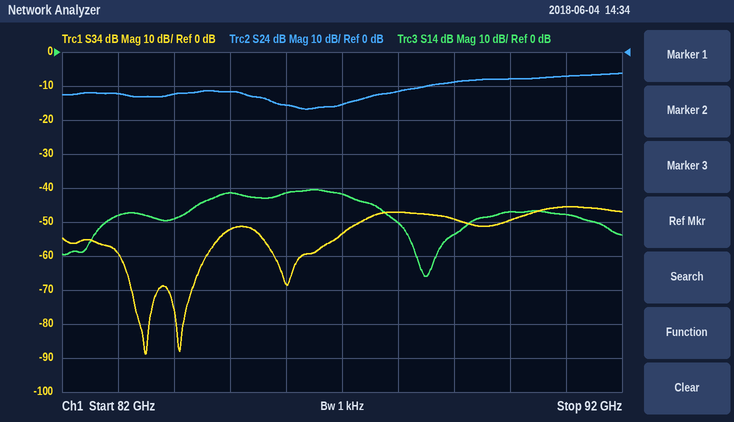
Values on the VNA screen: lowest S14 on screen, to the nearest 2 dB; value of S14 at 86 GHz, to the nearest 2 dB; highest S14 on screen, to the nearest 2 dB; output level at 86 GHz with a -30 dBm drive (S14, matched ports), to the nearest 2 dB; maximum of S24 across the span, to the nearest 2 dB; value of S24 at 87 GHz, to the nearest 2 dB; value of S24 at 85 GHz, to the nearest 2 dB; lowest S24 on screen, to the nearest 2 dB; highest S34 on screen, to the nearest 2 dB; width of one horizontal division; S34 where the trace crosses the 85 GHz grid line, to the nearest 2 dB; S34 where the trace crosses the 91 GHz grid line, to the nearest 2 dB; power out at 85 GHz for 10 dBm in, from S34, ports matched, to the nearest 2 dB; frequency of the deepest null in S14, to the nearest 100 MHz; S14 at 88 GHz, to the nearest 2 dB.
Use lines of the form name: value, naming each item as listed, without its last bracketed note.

lowest S14 on screen, to the nearest 2 dB: -66 dB
value of S14 at 86 GHz, to the nearest 2 dB: -42 dB
highest S14 on screen, to the nearest 2 dB: -40 dB
output level at 86 GHz with a -30 dBm drive (S14, matched ports), to the nearest 2 dB: -72 dBm
maximum of S24 across the span, to the nearest 2 dB: -6 dB
value of S24 at 87 GHz, to the nearest 2 dB: -16 dB
value of S24 at 85 GHz, to the nearest 2 dB: -12 dB
lowest S24 on screen, to the nearest 2 dB: -16 dB
highest S34 on screen, to the nearest 2 dB: -46 dB
width of one horizontal division: 1 GHz
S34 where the trace crosses the 85 GHz grid line, to the nearest 2 dB: -52 dB
S34 where the trace crosses the 91 GHz grid line, to the nearest 2 dB: -46 dB
power out at 85 GHz for 10 dBm in, from S34, ports matched, to the nearest 2 dB: -42 dBm
frequency of the deepest null in S14, to the nearest 100 MHz: 88.5 GHz
S14 at 88 GHz, to the nearest 2 dB: -50 dB
